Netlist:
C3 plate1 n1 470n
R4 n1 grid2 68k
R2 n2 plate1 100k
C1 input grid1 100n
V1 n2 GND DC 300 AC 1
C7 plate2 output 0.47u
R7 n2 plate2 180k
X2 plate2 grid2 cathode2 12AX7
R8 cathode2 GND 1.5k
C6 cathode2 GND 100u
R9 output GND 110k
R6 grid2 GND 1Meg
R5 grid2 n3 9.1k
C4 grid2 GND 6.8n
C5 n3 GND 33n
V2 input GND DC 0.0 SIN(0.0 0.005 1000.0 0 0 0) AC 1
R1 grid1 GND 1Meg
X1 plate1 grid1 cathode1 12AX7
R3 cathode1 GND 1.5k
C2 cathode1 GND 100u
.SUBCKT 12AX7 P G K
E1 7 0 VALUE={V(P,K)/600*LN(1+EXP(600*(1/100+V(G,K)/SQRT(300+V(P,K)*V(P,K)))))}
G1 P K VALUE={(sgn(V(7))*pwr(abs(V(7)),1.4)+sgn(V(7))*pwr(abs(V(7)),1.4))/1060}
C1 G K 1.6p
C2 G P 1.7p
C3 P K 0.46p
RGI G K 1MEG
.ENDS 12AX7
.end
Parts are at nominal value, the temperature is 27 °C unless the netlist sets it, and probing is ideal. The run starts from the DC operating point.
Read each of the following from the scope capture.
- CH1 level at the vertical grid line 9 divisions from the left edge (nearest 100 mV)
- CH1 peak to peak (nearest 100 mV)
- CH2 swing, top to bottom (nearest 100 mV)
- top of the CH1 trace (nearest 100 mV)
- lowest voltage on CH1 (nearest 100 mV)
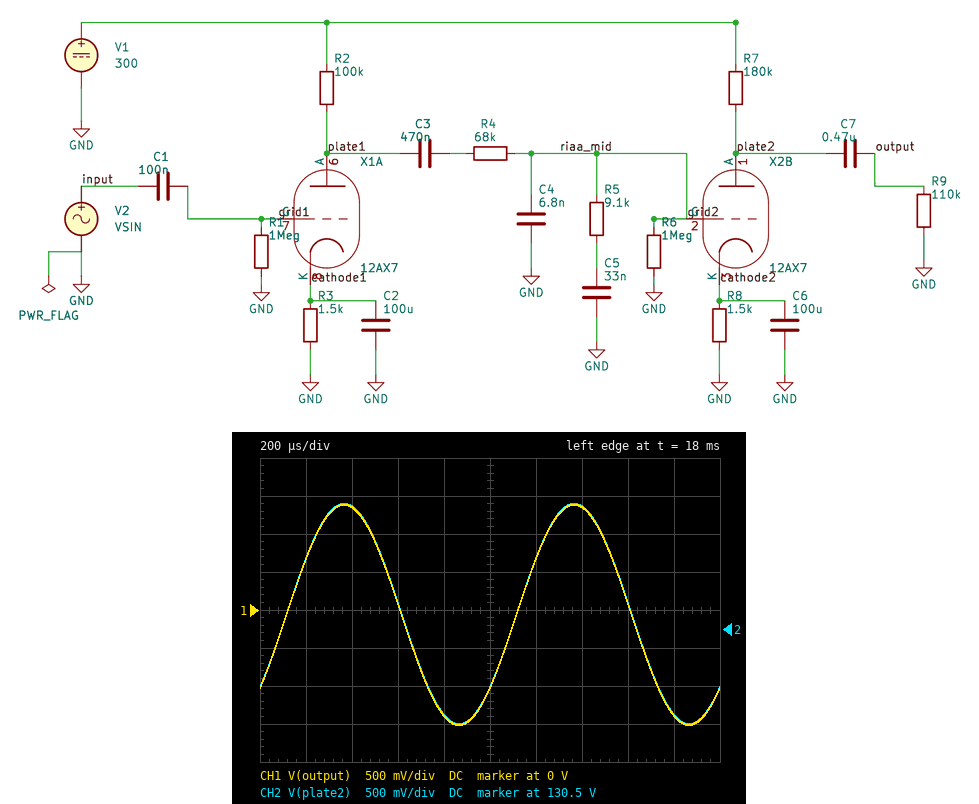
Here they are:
-1.4 V
2.9 V
2.9 V
1.4 V
-1.5 V
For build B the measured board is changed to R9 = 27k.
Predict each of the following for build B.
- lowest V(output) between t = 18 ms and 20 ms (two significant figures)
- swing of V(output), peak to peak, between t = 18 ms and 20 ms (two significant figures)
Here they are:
-850 mV
1.6 V
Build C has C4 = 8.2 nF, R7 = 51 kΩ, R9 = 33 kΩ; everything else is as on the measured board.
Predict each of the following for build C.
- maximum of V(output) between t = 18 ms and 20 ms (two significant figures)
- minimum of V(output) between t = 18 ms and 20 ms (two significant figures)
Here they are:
730 mV
-810 mV
